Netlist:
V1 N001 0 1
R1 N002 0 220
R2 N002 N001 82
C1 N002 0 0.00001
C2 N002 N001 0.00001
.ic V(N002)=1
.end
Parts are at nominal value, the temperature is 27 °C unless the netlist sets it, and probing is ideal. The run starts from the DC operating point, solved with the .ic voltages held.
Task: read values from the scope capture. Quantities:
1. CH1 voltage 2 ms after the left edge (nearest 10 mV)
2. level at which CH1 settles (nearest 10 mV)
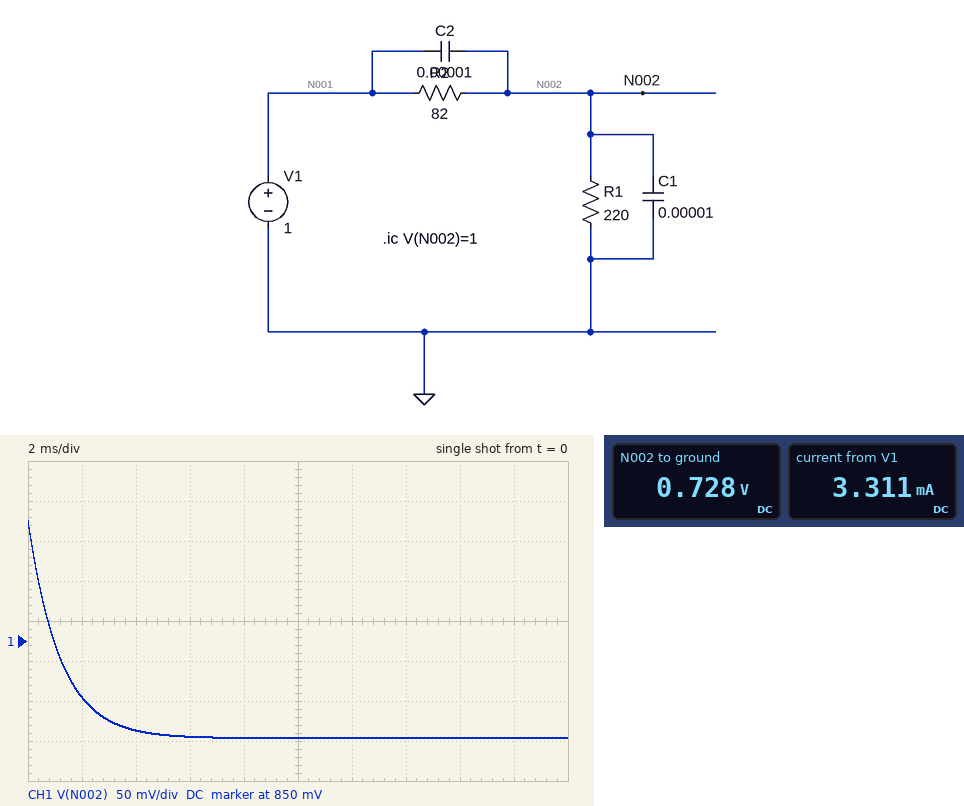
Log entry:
780 mV
730 mV
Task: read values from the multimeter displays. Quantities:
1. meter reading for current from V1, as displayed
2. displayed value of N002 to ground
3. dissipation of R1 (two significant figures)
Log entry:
3.311 mA
0.728 V
2.4 mW
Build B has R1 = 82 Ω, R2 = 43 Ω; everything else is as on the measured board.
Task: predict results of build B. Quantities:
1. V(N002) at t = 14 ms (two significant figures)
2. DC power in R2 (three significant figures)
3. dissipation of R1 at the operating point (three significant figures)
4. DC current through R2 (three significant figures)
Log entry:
660 mV
2.75 mW
5.25 mW
8.00 mA
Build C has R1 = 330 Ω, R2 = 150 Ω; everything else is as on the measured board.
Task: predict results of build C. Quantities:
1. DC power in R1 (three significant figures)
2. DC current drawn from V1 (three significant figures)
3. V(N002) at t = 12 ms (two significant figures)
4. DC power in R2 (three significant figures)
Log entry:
1.43 mW
2.08 mA
690 mV
651 µW
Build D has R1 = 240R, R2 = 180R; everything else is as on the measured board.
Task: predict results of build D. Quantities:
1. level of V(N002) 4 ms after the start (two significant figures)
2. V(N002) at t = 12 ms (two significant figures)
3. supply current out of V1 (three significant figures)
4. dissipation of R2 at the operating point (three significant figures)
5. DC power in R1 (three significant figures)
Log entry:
630 mV
570 mV
2.38 mA
1.02 mW
1.36 mW
